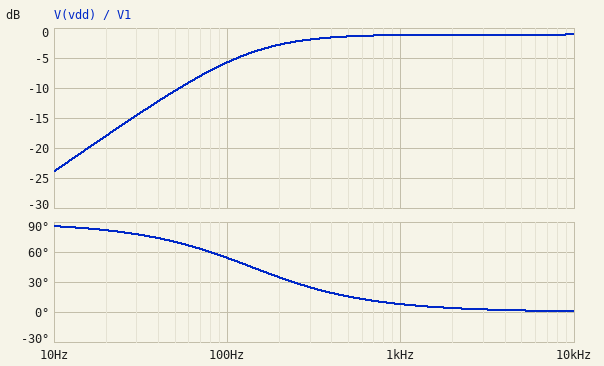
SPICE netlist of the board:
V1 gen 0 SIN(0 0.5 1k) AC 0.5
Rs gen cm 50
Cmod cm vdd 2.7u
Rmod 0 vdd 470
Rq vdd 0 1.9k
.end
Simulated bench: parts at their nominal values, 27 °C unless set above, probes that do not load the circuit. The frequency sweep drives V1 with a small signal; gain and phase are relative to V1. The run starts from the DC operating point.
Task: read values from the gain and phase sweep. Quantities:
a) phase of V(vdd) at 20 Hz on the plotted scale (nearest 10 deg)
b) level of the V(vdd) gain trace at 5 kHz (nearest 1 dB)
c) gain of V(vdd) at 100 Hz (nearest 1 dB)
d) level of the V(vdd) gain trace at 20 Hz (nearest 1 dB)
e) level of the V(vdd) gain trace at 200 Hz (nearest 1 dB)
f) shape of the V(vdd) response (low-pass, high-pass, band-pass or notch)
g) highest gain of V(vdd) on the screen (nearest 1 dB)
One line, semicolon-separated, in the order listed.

80 deg; -1 dB; -6 dB; -18 dB; -3 dB; high-pass; -1 dB
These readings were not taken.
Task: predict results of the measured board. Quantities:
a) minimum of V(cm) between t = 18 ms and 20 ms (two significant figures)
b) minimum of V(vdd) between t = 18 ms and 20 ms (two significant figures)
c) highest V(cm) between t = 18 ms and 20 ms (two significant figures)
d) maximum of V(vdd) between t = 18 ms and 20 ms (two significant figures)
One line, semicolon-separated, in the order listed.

-440 mV; -440 mV; 440 mV; 440 mV
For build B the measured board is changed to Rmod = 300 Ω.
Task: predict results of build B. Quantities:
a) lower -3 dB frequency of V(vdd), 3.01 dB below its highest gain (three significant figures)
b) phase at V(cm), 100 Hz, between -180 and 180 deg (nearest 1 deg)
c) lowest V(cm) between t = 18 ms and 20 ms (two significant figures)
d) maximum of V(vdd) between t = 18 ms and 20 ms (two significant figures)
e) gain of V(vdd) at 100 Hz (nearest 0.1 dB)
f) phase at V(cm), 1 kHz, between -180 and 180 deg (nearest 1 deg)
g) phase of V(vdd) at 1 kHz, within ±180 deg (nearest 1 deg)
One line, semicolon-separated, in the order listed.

191 Hz; -4 deg; -420 mV; 410 mV; -8.2 dB; -2 deg; 11 deg
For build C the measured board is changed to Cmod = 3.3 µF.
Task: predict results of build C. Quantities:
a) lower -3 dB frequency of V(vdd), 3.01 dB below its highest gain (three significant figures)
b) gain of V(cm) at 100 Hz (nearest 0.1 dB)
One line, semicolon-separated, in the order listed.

113 Hz; -0.4 dB
